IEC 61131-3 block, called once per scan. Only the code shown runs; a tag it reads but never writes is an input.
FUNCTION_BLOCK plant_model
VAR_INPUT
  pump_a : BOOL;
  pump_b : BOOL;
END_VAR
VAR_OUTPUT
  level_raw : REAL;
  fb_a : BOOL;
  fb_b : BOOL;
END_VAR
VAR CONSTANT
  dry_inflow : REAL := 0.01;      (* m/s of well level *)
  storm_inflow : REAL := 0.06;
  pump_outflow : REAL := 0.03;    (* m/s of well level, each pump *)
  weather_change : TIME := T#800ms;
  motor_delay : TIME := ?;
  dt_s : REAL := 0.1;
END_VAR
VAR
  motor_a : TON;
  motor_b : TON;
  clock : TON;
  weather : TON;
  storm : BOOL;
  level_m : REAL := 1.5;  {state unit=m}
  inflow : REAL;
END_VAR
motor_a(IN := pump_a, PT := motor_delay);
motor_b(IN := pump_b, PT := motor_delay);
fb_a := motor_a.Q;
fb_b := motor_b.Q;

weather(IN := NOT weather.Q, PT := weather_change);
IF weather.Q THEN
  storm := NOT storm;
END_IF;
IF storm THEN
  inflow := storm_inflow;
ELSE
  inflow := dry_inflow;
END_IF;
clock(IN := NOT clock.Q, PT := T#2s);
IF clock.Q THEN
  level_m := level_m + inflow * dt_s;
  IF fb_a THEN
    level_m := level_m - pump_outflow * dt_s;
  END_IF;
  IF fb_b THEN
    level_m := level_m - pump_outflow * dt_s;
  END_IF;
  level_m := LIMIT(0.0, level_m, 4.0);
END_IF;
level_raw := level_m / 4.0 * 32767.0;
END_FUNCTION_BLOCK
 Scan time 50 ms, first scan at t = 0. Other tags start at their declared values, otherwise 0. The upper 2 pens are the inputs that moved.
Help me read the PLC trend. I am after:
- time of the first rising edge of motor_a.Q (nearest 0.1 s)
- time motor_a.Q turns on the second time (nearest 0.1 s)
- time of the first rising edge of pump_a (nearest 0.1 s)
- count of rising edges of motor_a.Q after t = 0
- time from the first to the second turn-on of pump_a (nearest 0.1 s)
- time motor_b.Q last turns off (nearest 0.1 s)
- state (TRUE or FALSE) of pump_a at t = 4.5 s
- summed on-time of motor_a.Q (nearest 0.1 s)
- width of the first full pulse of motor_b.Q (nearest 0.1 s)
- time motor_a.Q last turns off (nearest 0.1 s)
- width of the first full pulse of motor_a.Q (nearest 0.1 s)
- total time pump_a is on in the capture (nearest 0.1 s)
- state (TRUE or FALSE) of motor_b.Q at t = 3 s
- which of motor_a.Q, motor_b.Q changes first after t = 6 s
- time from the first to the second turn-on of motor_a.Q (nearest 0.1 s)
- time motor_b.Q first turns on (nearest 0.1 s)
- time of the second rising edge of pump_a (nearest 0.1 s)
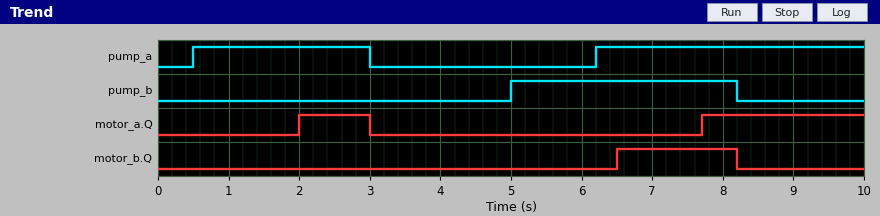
2.0 s
7.7 s
0.5 s
2
5.7 s
8.2 s
FALSE
3.3 s
1.7 s
3.0 s
1.0 s
6.3 s
FALSE
motor_b.Q
5.7 s
6.5 s
6.2 s
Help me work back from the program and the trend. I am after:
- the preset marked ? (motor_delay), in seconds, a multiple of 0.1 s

1.5 s
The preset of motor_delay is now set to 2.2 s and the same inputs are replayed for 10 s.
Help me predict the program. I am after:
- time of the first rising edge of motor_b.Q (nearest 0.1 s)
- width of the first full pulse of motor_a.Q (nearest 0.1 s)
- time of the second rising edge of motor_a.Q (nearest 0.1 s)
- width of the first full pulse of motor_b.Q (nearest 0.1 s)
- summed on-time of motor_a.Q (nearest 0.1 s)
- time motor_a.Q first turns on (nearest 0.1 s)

7.2 s
0.3 s
8.4 s
1.0 s
1.9 s
2.7 s
